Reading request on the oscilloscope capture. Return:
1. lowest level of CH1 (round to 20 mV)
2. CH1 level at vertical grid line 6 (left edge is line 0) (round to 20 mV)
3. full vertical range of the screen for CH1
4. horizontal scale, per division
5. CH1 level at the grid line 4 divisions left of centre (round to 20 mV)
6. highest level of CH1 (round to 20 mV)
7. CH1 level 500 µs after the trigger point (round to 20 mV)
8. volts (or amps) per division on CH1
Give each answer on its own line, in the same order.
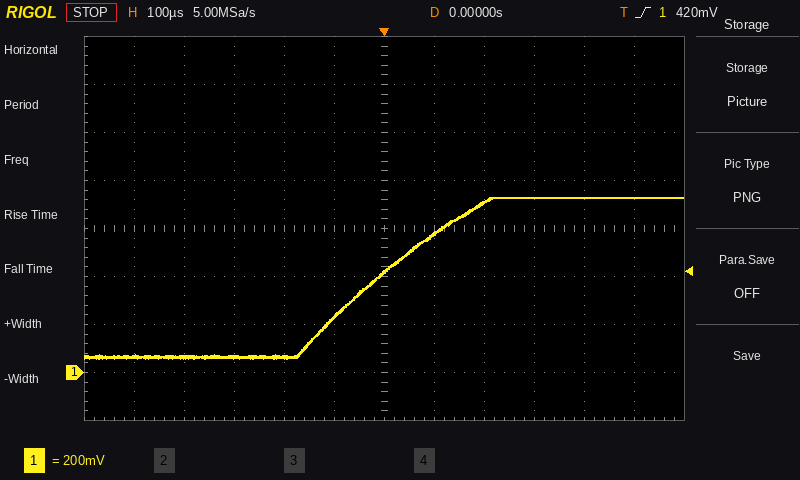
60 mV
420 mV
1.6 V
100 µs
60 mV
720 mV
720 mV
200 mV
